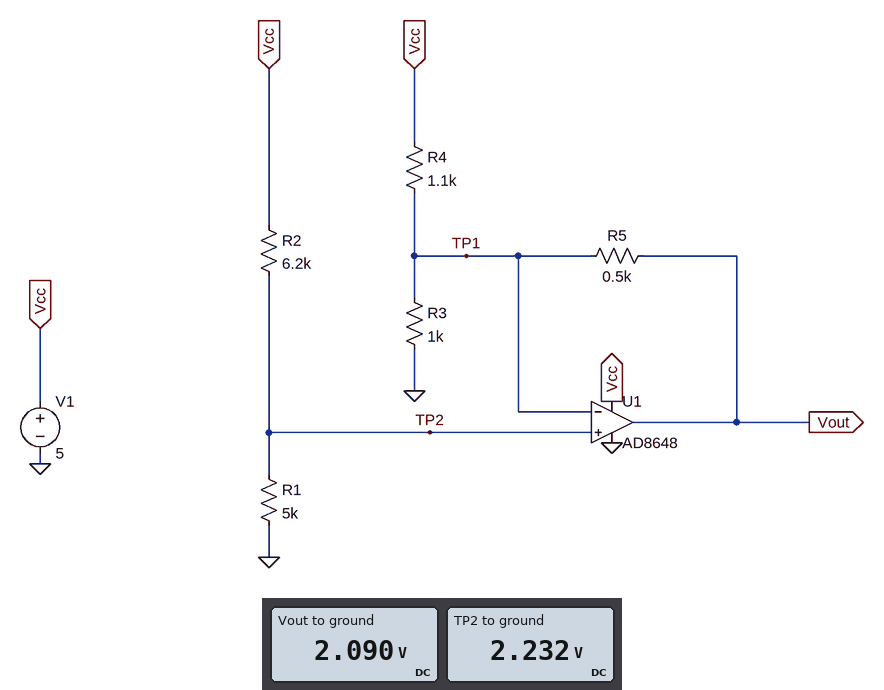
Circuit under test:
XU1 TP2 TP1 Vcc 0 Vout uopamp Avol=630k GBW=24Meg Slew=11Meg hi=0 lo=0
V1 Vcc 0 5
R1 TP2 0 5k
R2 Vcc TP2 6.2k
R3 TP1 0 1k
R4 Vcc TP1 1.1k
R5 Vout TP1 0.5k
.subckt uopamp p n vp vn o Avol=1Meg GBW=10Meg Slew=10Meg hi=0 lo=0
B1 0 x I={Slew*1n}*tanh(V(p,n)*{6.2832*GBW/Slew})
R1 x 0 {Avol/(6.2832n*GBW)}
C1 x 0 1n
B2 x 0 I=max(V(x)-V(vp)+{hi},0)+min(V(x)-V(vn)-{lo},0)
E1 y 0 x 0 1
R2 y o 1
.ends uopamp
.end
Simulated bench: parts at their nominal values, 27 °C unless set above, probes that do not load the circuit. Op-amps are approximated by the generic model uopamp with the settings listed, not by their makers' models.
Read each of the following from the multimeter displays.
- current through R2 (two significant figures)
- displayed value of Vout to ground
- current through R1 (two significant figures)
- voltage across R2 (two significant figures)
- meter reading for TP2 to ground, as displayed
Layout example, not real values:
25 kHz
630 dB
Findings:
450 µA
2.090 V
450 µA
2.8 V
2.232 V
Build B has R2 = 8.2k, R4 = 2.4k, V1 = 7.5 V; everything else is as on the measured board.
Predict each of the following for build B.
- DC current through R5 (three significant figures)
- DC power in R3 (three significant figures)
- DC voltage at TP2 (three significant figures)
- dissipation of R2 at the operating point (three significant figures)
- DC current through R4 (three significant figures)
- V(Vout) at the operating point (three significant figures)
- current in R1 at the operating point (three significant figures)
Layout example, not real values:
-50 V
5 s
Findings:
900 µA
8.07 mW
2.84 V
2.65 mW
1.94 mA
3.29 V
568 µA
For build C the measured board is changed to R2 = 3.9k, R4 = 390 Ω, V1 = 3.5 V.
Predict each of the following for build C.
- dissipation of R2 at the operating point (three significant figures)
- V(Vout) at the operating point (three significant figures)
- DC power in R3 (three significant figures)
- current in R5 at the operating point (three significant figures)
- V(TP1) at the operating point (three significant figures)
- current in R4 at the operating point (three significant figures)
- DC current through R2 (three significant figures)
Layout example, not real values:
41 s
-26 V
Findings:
603 µW
983 mV
3.87 mW
1.97 mA
1.97 V
3.93 mA
393 µA
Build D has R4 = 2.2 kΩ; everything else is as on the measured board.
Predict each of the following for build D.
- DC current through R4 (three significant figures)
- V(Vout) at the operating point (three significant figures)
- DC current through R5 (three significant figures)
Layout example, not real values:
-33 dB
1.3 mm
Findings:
1.26 mA
2.72 V
974 µA
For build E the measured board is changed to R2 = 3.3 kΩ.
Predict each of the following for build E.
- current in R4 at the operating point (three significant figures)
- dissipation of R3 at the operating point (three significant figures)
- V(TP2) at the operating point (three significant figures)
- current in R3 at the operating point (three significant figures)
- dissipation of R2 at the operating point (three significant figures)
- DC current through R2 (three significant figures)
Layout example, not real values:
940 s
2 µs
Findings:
1.81 mA
9.07 mW
3.01 V
3.01 mA
1.20 mW
602 µA
